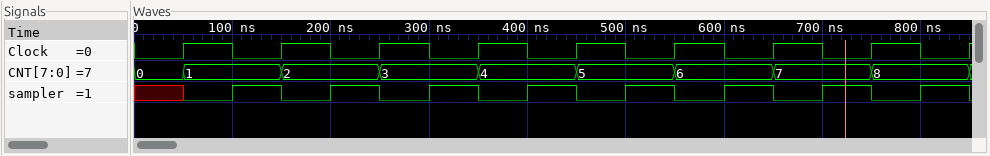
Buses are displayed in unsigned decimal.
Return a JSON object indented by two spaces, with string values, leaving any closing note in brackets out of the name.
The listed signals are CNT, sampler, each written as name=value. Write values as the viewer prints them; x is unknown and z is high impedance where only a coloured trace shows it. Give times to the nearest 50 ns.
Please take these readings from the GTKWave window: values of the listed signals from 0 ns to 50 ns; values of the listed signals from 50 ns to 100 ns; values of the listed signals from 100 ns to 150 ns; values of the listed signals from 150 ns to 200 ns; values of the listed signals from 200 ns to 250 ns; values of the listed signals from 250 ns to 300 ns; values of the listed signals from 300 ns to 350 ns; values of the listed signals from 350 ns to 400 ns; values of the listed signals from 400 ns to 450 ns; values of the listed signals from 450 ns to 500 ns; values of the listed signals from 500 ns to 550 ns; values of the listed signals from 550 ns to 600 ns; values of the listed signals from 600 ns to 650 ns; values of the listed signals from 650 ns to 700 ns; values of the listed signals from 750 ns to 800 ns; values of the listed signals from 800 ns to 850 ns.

{
  "values of the listed signals from 0 ns to 50 ns": "CNT=0, sampler=x",
  "values of the listed signals from 50 ns to 100 ns": "CNT=1, sampler=0",
  "values of the listed signals from 100 ns to 150 ns": "CNT=1, sampler=1",
  "values of the listed signals from 150 ns to 200 ns": "CNT=2, sampler=0",
  "values of the listed signals from 200 ns to 250 ns": "CNT=2, sampler=1",
  "values of the listed signals from 250 ns to 300 ns": "CNT=3, sampler=0",
  "values of the listed signals from 300 ns to 350 ns": "CNT=3, sampler=1",
  "values of the listed signals from 350 ns to 400 ns": "CNT=4, sampler=0",
  "values of the listed signals from 400 ns to 450 ns": "CNT=4, sampler=1",
  "values of the listed signals from 450 ns to 500 ns": "CNT=5, sampler=0",
  "values of the listed signals from 500 ns to 550 ns": "CNT=5, sampler=1",
  "values of the listed signals from 550 ns to 600 ns": "CNT=6, sampler=0",
  "values of the listed signals from 600 ns to 650 ns": "CNT=6, sampler=1",
  "values of the listed signals from 650 ns to 700 ns": "CNT=7, sampler=0",
  "values of the listed signals from 750 ns to 800 ns": "CNT=8, sampler=0",
  "values of the listed signals from 800 ns to 850 ns": "CNT=8, sampler=1"
}
